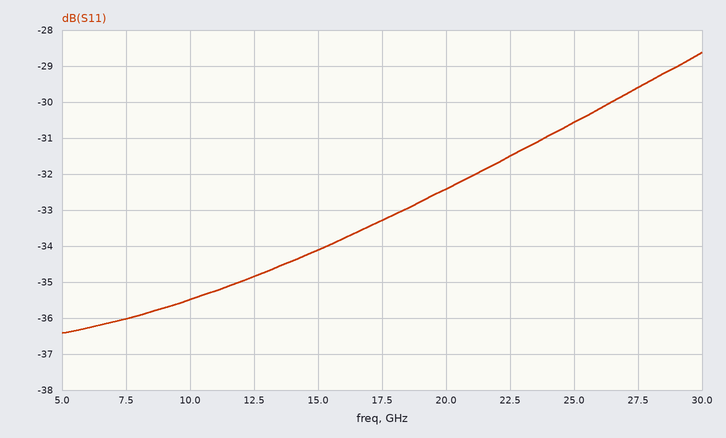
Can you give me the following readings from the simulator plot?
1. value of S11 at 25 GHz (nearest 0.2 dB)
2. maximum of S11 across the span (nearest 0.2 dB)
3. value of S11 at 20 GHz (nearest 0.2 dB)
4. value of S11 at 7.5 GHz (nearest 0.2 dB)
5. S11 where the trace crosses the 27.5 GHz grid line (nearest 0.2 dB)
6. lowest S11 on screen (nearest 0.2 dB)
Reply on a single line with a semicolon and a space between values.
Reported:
-30.6 dB; -28.6 dB; -32.4 dB; -36.0 dB; -29.6 dB; -36.4 dB
